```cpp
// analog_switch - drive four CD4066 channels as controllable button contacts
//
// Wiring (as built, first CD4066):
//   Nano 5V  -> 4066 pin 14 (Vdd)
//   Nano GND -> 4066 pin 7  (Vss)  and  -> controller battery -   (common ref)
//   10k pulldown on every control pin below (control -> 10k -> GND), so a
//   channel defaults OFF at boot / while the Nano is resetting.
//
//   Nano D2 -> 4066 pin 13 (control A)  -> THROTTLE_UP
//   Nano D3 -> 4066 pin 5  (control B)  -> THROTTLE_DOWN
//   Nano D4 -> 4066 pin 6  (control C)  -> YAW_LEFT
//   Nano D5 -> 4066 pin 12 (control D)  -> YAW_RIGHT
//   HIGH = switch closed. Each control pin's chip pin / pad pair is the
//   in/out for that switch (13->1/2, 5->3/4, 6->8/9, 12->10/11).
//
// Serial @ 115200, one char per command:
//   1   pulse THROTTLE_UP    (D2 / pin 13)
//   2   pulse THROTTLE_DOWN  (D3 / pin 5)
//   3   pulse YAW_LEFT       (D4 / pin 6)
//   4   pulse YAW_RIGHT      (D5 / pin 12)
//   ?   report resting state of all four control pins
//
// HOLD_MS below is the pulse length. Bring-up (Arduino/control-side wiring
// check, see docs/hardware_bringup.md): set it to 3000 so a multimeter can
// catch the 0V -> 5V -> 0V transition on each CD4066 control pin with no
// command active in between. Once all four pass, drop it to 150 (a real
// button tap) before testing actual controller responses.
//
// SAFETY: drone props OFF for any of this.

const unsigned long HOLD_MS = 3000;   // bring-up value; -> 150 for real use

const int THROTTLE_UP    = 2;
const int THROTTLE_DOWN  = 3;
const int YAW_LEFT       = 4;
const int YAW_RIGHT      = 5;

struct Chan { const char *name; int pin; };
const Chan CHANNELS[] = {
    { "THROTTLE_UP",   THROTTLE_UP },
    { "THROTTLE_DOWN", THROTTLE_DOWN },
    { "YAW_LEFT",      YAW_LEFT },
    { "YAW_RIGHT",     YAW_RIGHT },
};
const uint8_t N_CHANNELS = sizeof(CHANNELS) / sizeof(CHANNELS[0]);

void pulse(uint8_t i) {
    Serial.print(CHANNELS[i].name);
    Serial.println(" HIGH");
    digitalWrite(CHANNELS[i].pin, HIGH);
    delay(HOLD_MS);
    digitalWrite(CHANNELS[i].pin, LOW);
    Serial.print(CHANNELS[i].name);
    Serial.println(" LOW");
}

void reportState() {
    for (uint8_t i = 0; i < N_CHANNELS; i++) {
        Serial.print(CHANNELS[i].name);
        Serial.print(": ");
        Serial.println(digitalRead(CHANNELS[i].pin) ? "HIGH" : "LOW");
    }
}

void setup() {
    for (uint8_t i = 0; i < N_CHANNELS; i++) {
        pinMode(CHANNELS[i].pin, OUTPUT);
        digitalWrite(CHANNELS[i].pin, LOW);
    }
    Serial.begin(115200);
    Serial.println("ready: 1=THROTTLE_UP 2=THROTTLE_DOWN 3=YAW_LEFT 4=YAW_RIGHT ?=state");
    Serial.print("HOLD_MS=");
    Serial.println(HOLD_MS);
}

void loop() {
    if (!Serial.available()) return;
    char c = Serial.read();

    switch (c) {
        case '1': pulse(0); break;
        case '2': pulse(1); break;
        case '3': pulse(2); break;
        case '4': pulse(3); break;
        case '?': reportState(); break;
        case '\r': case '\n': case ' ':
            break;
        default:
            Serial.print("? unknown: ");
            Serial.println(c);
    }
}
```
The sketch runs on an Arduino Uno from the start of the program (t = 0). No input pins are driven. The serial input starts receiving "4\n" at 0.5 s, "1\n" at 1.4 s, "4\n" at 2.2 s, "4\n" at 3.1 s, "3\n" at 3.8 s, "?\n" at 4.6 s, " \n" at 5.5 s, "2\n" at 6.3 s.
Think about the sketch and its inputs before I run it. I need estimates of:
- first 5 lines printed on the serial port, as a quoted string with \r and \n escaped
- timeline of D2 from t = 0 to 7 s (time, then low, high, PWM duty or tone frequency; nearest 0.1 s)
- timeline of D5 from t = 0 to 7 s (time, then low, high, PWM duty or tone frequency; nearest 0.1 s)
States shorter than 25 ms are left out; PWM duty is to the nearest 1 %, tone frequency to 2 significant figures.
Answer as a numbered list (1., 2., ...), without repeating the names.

1. "ready: 1=THROTTLE_UP 2=THROTTLE_DOWN 3=YAW_LEFT 4=YAW_RIGHT ?=state\r\nHOLD_MS=3000\r\nYAW_RIGHT HIGH\r\nYAW_RIGHT LOW\r\nTHROTTLE_UP HIGH\r\n"
2. 0 s low; 3.5 s high; 6.5 s low
3. 0 s low; 0.5 s high; 3.5 s low; 6.5 s high
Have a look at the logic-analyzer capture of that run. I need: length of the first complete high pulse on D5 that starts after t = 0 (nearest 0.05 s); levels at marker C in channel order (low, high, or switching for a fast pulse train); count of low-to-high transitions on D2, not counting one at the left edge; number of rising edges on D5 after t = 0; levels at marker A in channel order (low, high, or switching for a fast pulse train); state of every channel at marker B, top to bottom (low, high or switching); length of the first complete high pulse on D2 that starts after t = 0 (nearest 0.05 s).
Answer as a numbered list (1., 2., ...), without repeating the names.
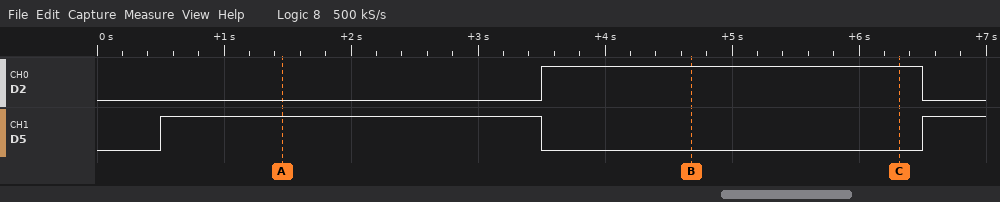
1. 3.00 s
2. D2 high, D5 low
3. 1
4. 2
5. D2 low, D5 high
6. D2 high, D5 low
7. 3.00 s
